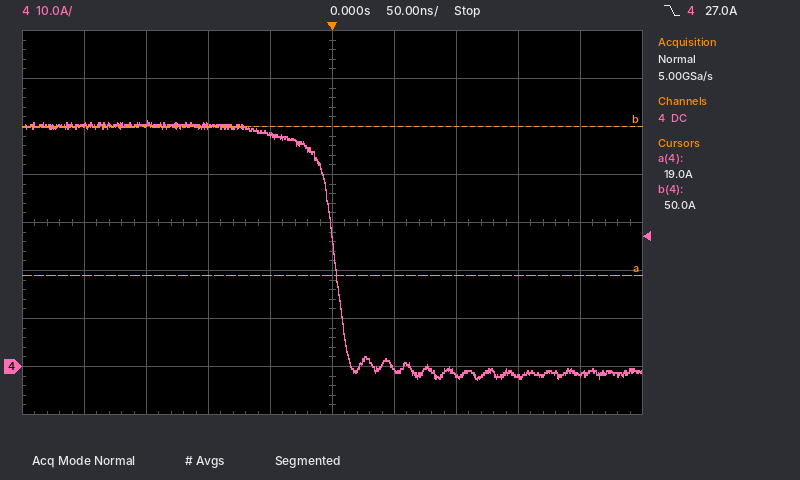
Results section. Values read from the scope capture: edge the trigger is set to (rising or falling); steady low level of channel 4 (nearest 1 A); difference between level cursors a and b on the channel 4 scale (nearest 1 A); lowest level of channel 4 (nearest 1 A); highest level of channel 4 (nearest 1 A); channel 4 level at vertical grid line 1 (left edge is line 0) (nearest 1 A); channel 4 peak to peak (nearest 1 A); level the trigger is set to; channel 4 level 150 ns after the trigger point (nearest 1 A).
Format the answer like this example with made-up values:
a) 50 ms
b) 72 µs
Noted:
a) falling
b) -1 A
c) 31 A
d) -3 A
e) 51 A
f) 50 A
g) 54 A
h) 27.0 A
i) -2 A
